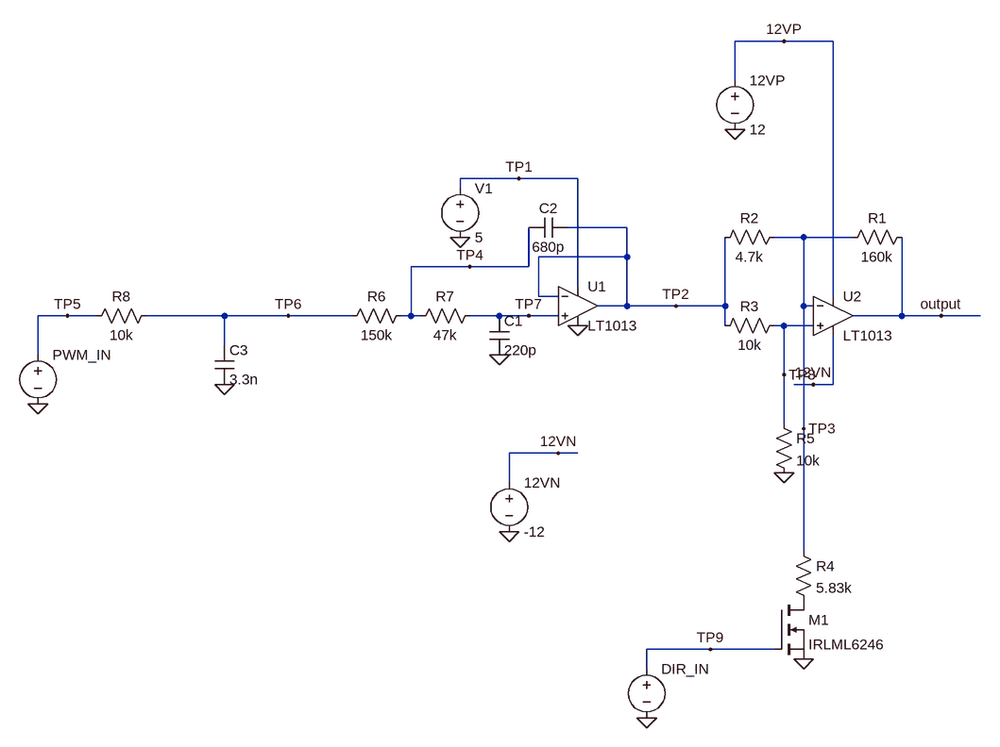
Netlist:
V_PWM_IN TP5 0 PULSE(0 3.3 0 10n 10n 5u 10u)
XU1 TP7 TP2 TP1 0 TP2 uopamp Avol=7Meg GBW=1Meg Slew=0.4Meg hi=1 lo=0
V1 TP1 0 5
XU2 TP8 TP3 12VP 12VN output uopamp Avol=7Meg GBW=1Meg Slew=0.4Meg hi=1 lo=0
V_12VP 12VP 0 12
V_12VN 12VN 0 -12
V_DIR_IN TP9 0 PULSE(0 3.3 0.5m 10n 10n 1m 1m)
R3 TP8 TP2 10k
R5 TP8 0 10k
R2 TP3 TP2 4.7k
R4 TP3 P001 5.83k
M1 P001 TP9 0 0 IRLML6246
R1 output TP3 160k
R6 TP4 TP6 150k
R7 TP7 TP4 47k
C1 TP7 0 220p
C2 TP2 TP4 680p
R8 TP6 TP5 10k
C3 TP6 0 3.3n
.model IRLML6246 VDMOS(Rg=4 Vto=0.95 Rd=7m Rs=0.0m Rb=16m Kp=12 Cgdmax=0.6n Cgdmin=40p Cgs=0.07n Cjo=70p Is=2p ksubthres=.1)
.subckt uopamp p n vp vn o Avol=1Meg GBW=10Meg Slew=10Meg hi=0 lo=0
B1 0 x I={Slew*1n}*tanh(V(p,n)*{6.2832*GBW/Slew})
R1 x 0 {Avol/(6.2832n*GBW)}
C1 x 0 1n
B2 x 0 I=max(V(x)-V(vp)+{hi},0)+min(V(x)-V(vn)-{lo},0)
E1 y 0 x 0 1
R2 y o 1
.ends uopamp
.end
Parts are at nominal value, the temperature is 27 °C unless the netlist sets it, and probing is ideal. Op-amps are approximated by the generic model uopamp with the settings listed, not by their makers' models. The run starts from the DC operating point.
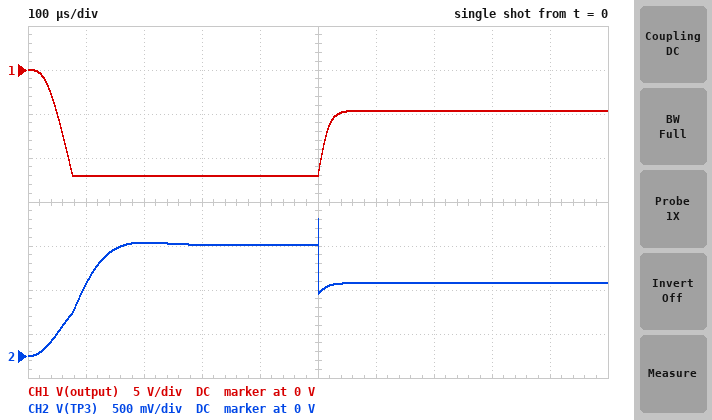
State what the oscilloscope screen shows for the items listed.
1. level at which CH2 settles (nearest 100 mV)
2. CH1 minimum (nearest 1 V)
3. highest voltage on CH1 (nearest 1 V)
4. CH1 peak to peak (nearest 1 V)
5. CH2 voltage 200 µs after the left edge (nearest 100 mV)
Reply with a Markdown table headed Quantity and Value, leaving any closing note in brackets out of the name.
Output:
| Quantity | Value |
|---|---|
| level at which CH2 settles | 800 mV |
| CH1 minimum | -12 V |
| highest voltage on CH1 | 0 V |
| CH1 peak to peak | 12 V |
| CH2 voltage 200 µs after the left edge | 1.3 V |
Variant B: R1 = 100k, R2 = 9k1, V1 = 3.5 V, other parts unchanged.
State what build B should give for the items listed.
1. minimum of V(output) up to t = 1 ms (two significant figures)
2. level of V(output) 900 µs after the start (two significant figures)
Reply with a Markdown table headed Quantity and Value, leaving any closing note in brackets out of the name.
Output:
| Quantity | Value |
|---|---|
| minimum of V(output) up to t = 1 ms | -8.4 V |
| level of V(output) 900 µs after the start | 5.9 V |
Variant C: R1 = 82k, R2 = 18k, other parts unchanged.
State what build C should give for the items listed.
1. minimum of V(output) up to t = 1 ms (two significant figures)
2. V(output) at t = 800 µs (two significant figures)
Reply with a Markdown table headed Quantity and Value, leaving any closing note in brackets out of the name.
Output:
| Quantity | Value |
|---|---|
| minimum of V(output) up to t = 1 ms | -3.0 V |
| V(output) at t = 800 µs | 8.7 V |
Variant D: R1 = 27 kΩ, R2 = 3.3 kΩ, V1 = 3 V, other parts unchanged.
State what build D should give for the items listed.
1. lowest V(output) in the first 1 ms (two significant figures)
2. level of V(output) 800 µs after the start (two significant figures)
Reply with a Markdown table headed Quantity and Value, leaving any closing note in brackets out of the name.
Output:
| Quantity | Value |
|---|---|
| lowest V(output) in the first 1 ms | -6.0 V |
| level of V(output) 800 µs after the start | -2.1 V |
